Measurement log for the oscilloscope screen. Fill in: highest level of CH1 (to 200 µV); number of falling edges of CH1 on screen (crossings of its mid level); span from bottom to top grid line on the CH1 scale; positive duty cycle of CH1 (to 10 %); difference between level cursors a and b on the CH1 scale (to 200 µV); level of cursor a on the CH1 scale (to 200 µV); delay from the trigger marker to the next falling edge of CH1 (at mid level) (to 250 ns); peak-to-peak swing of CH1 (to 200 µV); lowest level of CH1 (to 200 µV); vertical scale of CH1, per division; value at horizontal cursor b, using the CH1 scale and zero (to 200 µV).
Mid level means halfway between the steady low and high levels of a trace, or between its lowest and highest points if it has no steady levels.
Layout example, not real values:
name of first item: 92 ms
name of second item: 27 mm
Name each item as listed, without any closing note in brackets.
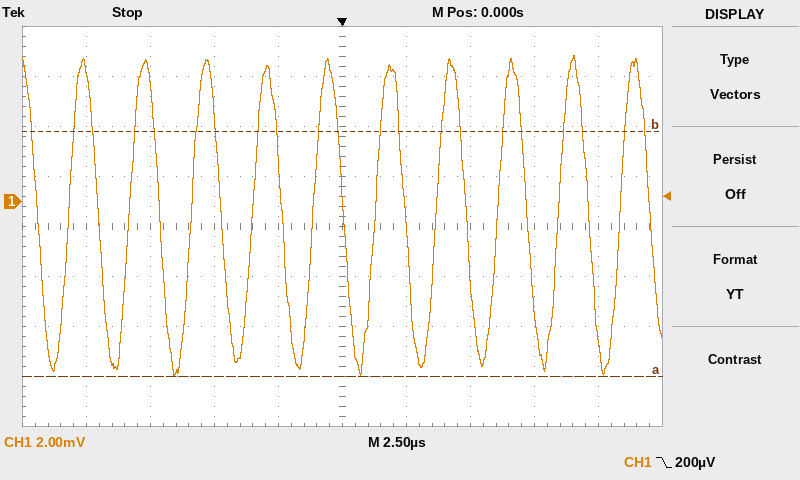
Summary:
highest level of CH1: 5.8 mV
number of falling edges of CH1 on screen: 11
span from bottom to top grid line on the CH1 scale: 16 mV
positive duty cycle of CH1: 50 %
difference between level cursors a and b on the CH1 scale: 9.8 mV
level of cursor a on the CH1 scale: -7.0 mV
delay from the trigger marker to the next falling edge of CH1 (at mid level): 2.50 µs
peak-to-peak swing of CH1: 12.8 mV
lowest level of CH1: -7.0 mV
vertical scale of CH1, per division: 2 mV
value at horizontal cursor b, using the CH1 scale and zero: 2.8 mV
